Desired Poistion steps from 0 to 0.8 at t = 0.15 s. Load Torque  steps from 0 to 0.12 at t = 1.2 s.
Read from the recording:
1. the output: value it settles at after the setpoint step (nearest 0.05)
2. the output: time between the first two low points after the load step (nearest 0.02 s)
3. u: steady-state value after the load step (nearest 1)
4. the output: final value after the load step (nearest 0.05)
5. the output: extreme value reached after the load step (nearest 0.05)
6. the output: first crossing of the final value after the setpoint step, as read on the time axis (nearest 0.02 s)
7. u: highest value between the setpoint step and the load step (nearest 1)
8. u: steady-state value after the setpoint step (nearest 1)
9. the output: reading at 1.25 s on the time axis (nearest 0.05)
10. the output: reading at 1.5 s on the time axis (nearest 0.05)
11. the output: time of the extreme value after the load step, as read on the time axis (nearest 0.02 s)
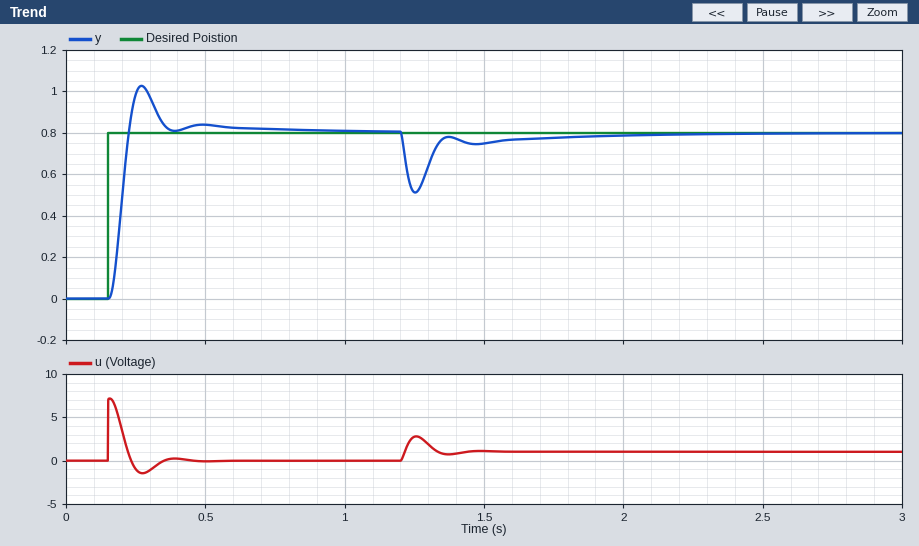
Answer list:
0.80
0.22 s
1
0.80
0.50
0.22 s
7
0
0.50
0.75
1.26 s
